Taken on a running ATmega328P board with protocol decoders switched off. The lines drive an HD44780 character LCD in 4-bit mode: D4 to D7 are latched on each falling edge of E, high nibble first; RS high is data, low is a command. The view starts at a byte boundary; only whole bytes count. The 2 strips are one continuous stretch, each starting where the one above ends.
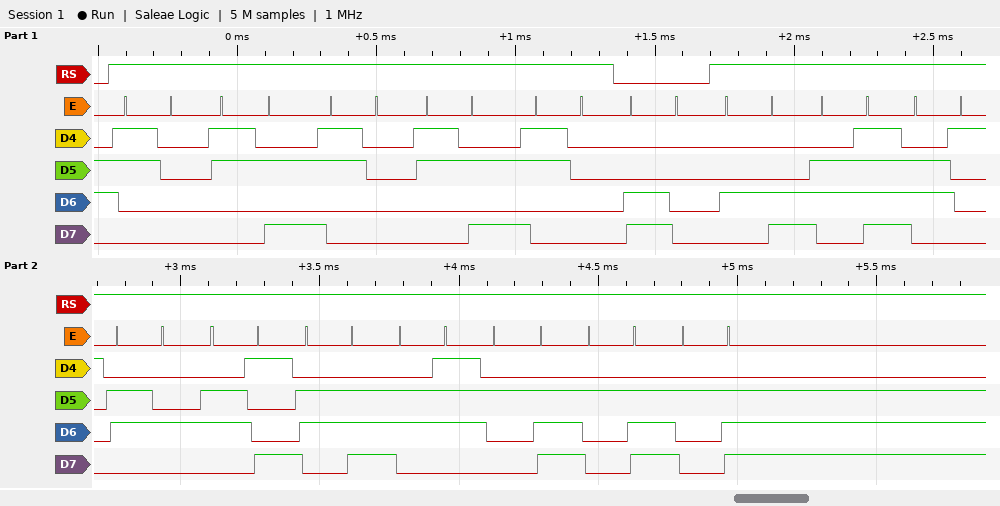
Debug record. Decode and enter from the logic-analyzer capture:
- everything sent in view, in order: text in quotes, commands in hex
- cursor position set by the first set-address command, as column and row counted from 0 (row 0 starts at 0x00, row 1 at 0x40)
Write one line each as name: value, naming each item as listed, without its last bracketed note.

everything sent in view, in order: text in quotes, commands in hex: "0:0:0" 0xC0 "Loading..."
cursor position set by the first set-address command, as column and row counted from 0: column 0, row 1
